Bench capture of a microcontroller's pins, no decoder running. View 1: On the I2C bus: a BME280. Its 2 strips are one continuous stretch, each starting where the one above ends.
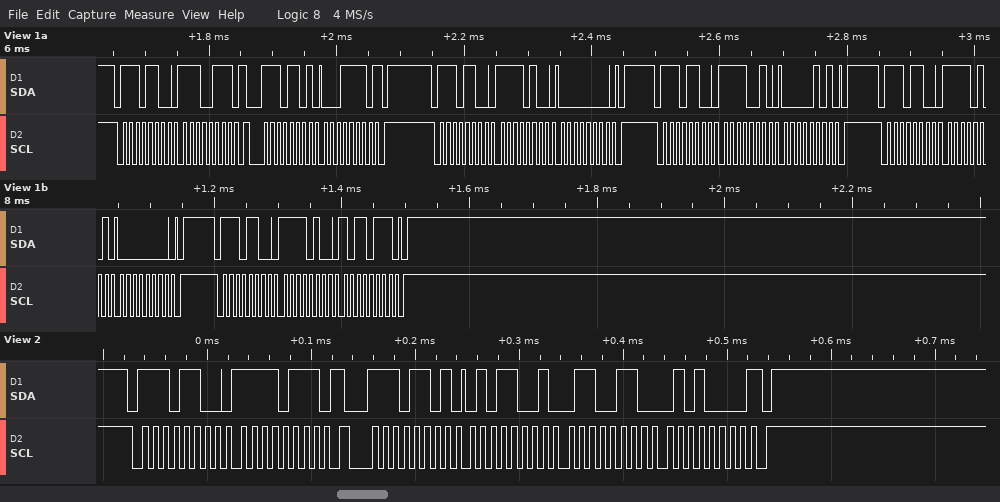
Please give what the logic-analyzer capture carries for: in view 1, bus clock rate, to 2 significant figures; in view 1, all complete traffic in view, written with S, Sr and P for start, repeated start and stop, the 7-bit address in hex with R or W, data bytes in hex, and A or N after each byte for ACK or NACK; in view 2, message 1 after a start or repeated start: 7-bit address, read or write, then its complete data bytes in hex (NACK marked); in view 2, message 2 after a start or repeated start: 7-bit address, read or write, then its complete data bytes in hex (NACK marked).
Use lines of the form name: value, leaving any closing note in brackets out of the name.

in view 1, bus clock rate, to 2 significant figures: 100 kHz
in view 1, all complete traffic in view, written with S, Sr and P for start, repeated start and stop, the 7-bit address in hex with R or W, data bytes in hex, and A or N after each byte for ACK or NACK: S 76W A E7 A Sr 76R A 1E N P S 76W A F4 A 00 A P S 76W A F2 A 05 A P S 76W A F5 A 00 A P S 76W A F4 A B7 A P
in view 2, message 1 after a start or repeated start: 7-bit address, read or write, then its complete data bytes in hex: 0x76 write: F7
in view 2, message 2 after a start or repeated start: 7-bit address, read or write, then its complete data bytes in hex: 0x76 read: 59 66 50 NACK
